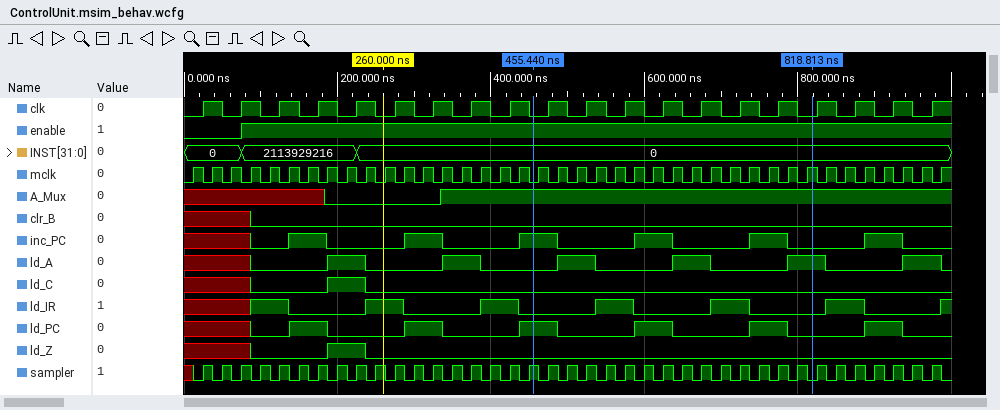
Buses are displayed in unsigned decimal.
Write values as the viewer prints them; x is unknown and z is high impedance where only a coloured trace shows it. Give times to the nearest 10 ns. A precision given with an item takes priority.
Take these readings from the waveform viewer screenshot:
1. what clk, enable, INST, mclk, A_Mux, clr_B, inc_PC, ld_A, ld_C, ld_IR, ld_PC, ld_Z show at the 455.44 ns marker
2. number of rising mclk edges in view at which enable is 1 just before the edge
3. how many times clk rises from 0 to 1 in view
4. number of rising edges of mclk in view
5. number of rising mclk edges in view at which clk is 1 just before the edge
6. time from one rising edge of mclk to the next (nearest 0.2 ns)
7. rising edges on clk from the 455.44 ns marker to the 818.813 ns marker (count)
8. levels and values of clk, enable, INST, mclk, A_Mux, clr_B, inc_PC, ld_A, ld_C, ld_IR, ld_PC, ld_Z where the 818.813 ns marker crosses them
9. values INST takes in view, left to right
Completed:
clk=0, enable=1, INST=0, mclk=0, A_Mux=1, clr_B=0, inc_PC=1, ld_A=0, ld_C=0, ld_IR=0, ld_PC=1, ld_Z=0
37
20
40
20
25 ns
7
clk=0, enable=1, INST=0, mclk=1, A_Mux=1, clr_B=0, inc_PC=0, ld_A=1, ld_C=0, ld_IR=0, ld_PC=0, ld_Z=0
0, 2113929216, 0
